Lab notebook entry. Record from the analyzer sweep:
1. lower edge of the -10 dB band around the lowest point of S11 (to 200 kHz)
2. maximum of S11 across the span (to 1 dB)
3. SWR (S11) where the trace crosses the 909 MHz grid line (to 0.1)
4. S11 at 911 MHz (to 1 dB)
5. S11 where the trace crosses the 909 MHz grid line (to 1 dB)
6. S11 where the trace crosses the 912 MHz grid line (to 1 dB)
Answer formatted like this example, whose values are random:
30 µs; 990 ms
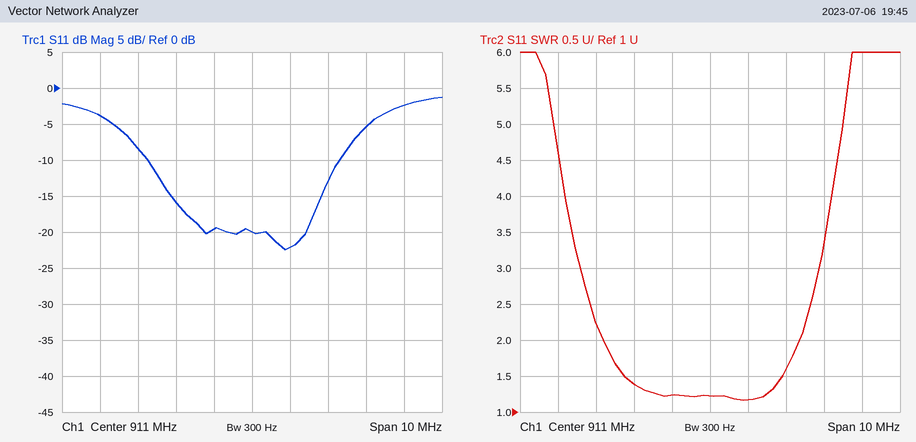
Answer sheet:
908.2 MHz; -1 dB; 1.4; -20 dB; -16 dB; -22 dB
